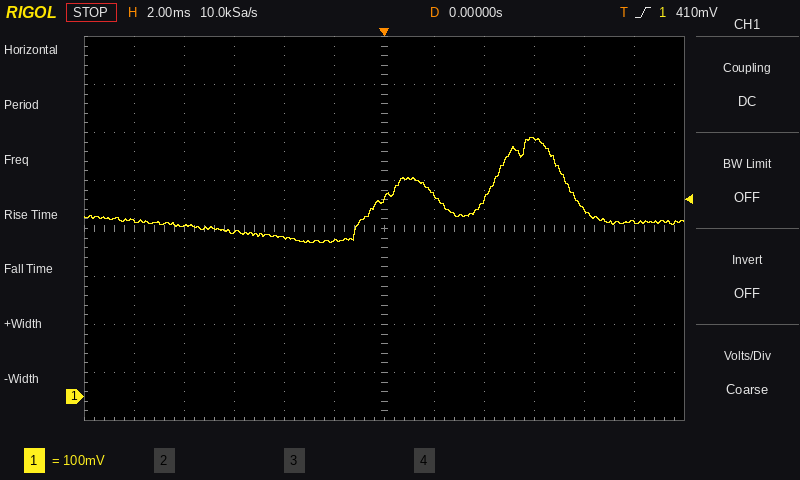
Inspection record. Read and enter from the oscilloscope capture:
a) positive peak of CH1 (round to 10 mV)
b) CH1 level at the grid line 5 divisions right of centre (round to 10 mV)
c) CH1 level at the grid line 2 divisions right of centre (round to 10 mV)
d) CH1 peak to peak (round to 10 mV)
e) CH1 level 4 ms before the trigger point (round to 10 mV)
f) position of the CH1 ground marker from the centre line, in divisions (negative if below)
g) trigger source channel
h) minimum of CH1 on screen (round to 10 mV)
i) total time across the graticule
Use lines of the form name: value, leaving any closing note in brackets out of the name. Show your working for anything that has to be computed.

positive peak of CH1: 540 mV
CH1 level at the grid line 5 divisions right of centre: 360 mV
CH1 level at the grid line 2 divisions right of centre: 410 mV
CH1 peak to peak: 540 mV − (320 mV) = 220 mV
CH1 level 4 ms before the trigger point: 330 mV
position of the CH1 ground marker from the centre line, in divisions: -3.5 div
trigger source channel: CH1
minimum of CH1 on screen: 320 mV
total time across the graticule: 24 ms
